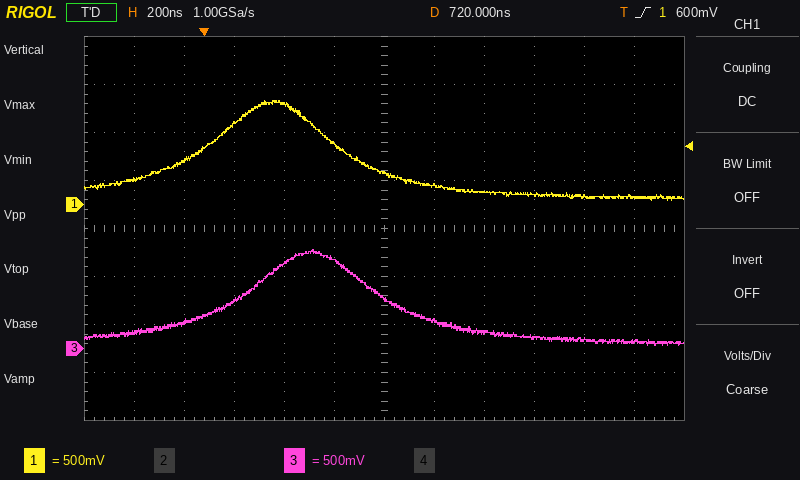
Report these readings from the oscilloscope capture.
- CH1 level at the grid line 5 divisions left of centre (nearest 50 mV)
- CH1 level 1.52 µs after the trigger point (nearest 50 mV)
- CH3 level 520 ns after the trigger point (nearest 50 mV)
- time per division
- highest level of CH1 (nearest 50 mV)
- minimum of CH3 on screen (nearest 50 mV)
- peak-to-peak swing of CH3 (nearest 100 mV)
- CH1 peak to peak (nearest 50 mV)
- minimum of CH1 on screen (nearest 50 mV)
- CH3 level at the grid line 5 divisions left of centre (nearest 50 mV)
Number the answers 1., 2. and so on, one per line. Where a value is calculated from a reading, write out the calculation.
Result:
1. 250 mV
2. 100 mV
3. 900 mV
4. 200 ns
5. 1.10 V
6. 50 mV
7. 1.00 V
8. 1.10 V − (50 mV) = 1.05 V
9. 50 mV
10. 150 mV
